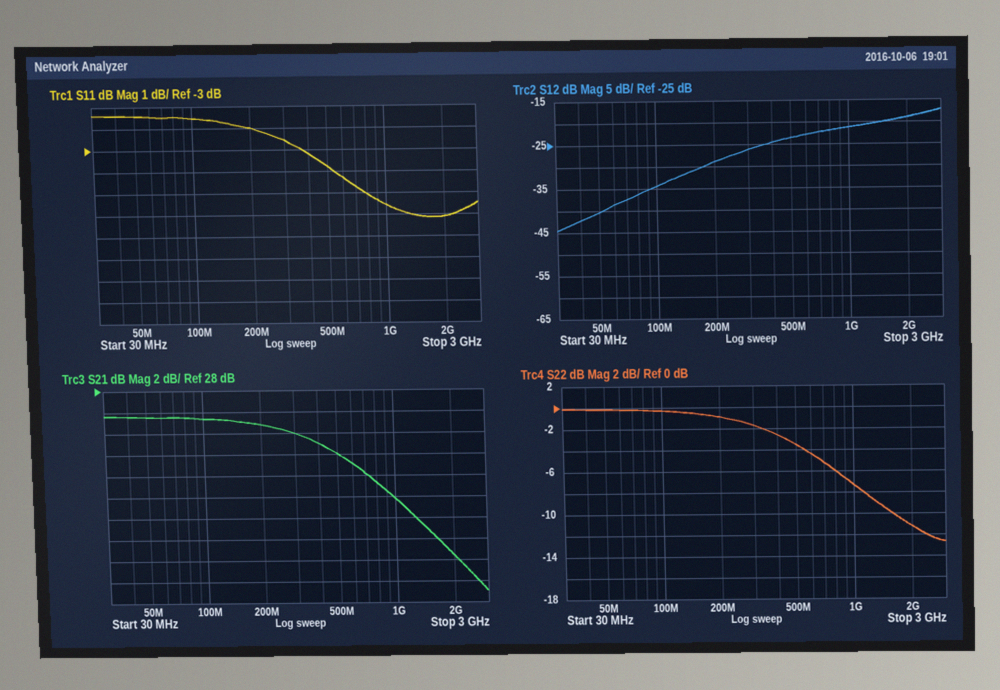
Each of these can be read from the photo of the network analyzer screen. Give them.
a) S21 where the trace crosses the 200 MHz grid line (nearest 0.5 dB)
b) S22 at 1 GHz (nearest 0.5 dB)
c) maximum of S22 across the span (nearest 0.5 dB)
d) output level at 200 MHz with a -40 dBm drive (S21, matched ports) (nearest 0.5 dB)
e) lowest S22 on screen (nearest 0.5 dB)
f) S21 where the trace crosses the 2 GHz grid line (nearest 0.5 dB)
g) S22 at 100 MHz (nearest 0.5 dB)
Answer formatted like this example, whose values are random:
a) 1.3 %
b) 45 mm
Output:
a) 25.0 dB
b) -7.5 dB
c) 0.0 dB
d) -15.0 dBm
e) -12.5 dB
f) 12.5 dB
g) -0.5 dB
